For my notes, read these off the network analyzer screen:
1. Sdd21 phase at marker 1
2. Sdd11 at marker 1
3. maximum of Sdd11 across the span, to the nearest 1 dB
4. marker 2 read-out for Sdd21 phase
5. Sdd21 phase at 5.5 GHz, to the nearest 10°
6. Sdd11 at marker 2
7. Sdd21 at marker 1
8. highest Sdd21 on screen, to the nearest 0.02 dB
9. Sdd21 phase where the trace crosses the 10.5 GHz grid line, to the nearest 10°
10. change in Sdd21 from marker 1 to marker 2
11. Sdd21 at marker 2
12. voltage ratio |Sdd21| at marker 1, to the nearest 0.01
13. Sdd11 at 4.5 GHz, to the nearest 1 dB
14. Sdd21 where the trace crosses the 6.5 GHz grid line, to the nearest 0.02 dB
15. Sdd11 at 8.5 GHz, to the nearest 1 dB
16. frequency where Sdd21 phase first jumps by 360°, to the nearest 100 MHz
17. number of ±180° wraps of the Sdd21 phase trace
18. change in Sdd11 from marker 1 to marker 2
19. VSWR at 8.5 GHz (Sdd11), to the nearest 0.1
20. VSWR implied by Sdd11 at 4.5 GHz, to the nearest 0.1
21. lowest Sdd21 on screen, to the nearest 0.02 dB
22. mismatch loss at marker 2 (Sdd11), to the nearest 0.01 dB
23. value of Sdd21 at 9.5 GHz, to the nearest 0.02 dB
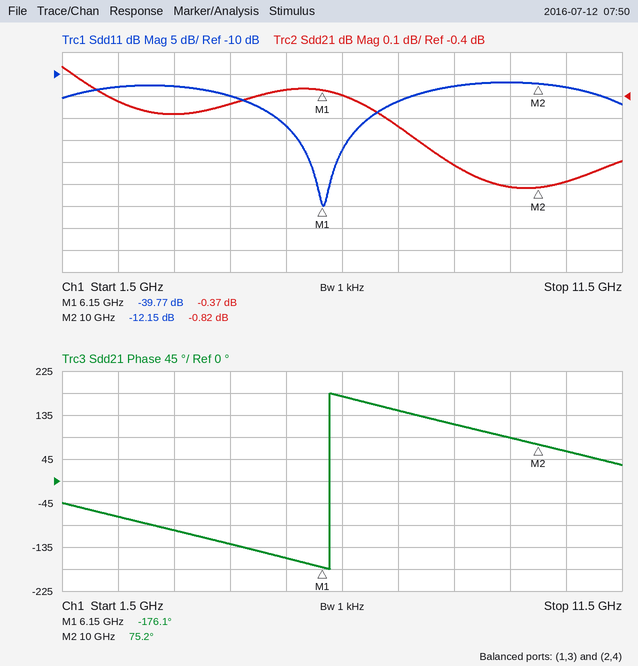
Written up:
-176.1°
-39.77 dB
-12 dB
75.2°
-160°
-12.15 dB
-0.37 dB
-0.26 dB
60°
-0.45 dB
-0.82 dB
0.96
-15 dB
-0.40 dB
-13 dB
6.3 GHz
1
27.62 dB
1.6
1.4
-0.82 dB
0.27 dB
-0.82 dB
